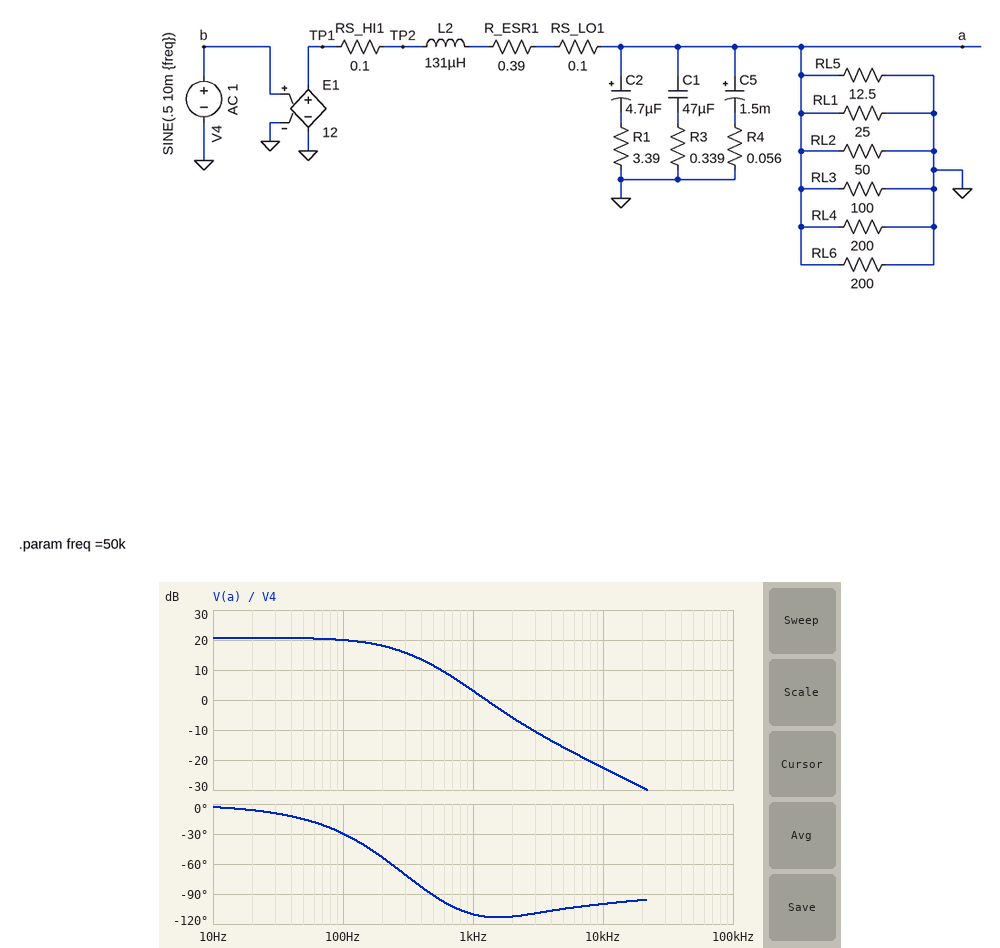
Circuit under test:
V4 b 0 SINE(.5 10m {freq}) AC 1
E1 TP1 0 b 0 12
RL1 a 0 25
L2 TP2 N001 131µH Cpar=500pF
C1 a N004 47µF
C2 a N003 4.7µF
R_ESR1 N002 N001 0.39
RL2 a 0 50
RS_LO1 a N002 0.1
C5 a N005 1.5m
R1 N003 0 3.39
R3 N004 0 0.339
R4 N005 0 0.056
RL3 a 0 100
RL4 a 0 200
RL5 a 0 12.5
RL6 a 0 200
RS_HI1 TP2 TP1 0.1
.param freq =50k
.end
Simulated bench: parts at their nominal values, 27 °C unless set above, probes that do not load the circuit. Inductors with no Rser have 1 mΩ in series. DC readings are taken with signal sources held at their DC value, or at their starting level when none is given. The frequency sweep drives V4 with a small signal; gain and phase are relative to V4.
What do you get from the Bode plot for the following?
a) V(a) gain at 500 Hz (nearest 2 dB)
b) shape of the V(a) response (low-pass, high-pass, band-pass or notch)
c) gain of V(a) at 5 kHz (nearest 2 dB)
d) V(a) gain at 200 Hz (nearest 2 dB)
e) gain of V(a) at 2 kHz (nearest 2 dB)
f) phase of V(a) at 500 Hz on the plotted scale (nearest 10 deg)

12 dB
low-pass
-16 dB
18 dB
-6 dB
-90 deg
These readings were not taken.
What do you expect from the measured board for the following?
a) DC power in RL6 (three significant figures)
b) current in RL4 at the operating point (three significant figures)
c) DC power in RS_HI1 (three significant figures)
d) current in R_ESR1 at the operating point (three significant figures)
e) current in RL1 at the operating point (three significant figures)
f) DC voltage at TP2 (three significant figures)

150 mW
27.4 mA
76.9 mW
877 mA
219 mA
5.91 V
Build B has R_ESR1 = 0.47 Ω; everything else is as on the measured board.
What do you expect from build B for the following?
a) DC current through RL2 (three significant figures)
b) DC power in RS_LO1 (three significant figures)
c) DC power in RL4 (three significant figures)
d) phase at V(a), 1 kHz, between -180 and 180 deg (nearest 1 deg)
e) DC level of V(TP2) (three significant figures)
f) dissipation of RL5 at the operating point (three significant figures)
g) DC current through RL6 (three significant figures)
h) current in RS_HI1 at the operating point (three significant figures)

108 mA
75.2 mW
147 mW
-107 deg
5.91 V
2.35 W
27.1 mA
867 mA
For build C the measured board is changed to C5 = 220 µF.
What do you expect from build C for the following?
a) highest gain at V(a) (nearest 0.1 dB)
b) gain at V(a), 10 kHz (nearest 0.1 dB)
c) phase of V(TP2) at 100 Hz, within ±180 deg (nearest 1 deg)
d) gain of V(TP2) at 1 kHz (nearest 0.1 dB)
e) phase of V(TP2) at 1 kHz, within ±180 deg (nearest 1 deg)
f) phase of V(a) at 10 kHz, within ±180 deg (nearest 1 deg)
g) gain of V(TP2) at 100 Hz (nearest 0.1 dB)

22.1 dB
-19.2 dB
-1 deg
20.4 dB
3 deg
-136 deg
21.4 dB
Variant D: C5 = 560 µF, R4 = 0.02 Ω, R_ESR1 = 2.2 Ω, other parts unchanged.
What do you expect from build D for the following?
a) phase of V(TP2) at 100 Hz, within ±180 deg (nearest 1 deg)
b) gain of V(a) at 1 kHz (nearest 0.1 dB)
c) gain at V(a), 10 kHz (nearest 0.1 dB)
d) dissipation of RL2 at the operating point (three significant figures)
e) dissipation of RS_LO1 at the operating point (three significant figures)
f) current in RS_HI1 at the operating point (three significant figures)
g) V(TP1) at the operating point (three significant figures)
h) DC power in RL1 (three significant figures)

-1 deg
1.9 dB
-26.9 dB
376 mW
48.1 mW
694 mA
6.00 V
752 mW
